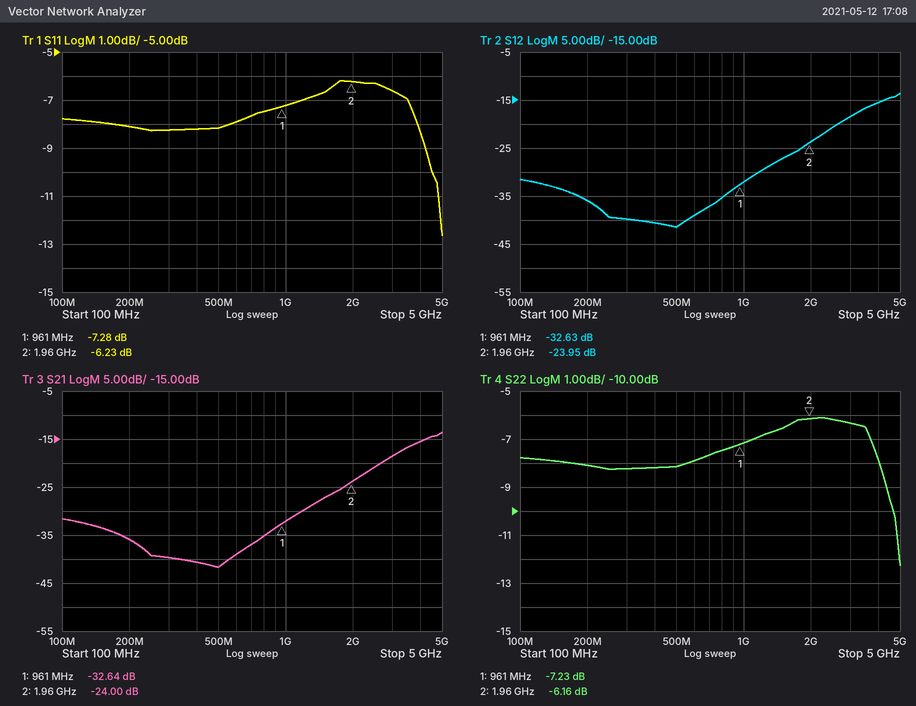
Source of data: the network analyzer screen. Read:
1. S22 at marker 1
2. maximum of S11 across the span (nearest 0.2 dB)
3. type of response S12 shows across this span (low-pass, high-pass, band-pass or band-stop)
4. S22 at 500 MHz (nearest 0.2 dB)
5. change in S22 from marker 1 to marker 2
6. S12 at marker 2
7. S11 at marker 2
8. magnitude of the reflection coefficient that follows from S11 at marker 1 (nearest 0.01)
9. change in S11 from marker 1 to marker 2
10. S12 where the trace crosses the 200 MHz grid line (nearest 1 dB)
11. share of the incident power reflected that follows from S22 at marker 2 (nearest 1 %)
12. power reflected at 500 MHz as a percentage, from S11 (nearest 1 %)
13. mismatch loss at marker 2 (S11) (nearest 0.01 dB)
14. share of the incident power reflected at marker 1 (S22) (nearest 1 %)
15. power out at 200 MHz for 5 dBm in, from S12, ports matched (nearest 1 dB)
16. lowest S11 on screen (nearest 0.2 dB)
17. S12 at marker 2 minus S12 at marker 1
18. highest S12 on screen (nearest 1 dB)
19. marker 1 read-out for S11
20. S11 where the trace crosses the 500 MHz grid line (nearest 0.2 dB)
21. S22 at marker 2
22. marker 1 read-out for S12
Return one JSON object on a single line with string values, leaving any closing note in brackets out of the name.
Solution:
{"S22 at marker 1": "-7.23 dB", "maximum of S11 across the span": "-6.2 dB", "type of response S12 shows across this span": "high-pass", "S22 at 500 MHz": "-8.2 dB", "change in S22 from marker 1 to marker 2": "1.07 dB", "S12 at marker 2": "-23.95 dB", "S11 at marker 2": "-6.23 dB", "magnitude of the reflection coefficient that follows from S11 at marker 1": "0.43", "change in S11 from marker 1 to marker 2": "1.05 dB", "S12 where the trace crosses the 200 MHz grid line": "-36 dB", "share of the incident power reflected that follows from S22 at marker 2": "24 %", "power reflected at 500 MHz as a percentage, from S11": "15 %", "mismatch loss at marker 2 (S11)": "1.18 dB", "share of the incident power reflected at marker 1 (S22)": "19 %", "power out at 200 MHz for 5 dBm in, from S12, ports matched": "-31 dBm", "lowest S11 on screen": "-12.6 dB", "S12 at marker 2 minus S12 at marker 1": "8.68 dB", "highest S12 on screen": "-14 dB", "marker 1 read-out for S11": "-7.28 dB", "S11 where the trace crosses the 500 MHz grid line": "-8.2 dB", "S22 at marker 2": "-6.16 dB", "marker 1 read-out for S12": "-32.63 dB"}
